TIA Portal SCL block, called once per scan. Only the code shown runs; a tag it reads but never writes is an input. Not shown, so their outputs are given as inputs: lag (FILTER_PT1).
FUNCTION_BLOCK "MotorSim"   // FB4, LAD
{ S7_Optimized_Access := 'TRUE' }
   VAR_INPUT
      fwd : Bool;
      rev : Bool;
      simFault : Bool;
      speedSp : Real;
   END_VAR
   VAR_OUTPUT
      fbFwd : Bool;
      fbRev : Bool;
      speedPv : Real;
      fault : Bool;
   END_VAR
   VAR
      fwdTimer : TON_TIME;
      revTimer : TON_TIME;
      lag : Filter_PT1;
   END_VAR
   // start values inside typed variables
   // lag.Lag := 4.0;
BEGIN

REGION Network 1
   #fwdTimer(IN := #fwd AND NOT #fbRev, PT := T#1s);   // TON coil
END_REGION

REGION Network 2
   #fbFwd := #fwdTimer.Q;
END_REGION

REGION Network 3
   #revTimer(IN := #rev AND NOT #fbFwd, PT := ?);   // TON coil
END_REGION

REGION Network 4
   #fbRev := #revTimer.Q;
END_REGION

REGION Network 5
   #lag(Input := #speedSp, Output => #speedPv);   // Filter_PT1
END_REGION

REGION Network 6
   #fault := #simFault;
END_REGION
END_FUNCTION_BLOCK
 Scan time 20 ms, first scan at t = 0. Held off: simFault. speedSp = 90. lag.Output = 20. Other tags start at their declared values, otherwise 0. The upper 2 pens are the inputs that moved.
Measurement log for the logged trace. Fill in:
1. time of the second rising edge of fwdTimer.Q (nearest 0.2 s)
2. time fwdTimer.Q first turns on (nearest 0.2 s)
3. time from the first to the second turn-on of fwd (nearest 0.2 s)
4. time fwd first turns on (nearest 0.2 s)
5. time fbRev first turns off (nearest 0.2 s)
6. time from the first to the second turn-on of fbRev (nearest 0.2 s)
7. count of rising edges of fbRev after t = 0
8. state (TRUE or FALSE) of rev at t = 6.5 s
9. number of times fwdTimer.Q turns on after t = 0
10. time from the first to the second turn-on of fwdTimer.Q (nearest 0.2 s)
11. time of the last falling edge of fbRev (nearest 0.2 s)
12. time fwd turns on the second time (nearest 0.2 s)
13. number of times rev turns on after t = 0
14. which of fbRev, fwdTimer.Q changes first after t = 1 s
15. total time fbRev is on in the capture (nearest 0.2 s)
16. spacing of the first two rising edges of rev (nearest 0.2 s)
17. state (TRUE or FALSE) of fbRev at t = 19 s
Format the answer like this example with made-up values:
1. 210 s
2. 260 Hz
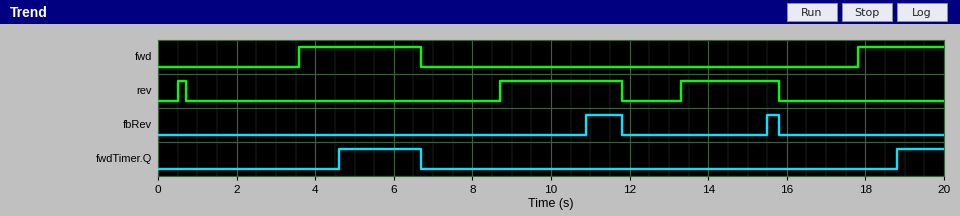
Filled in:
1. 18.8 s
2. 4.6 s
3. 14.2 s
4. 3.6 s
5. 11.8 s
6. 4.6 s
7. 2
8. FALSE
9. 2
10. 14.2 s
11. 15.8 s
12. 17.8 s
13. 3
14. fwdTimer.Q
15. 1.2 s
16. 8.2 s
17. FALSE
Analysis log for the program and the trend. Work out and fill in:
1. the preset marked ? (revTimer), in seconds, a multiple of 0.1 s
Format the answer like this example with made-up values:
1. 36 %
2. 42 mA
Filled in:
1. 2.2 s
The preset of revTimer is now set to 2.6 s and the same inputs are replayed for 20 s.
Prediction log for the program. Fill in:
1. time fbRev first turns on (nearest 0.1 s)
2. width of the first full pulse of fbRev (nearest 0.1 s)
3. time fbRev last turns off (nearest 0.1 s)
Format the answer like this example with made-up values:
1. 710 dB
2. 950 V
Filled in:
1. 11.3 s
2. 0.5 s
3. 11.8 s
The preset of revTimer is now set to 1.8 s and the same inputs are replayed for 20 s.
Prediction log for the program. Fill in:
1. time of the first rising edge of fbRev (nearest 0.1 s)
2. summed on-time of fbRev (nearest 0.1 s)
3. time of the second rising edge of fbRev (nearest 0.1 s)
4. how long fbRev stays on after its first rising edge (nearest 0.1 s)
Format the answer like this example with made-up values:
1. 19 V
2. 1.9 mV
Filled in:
1. 10.5 s
2. 2.0 s
3. 15.1 s
4. 1.3 s
